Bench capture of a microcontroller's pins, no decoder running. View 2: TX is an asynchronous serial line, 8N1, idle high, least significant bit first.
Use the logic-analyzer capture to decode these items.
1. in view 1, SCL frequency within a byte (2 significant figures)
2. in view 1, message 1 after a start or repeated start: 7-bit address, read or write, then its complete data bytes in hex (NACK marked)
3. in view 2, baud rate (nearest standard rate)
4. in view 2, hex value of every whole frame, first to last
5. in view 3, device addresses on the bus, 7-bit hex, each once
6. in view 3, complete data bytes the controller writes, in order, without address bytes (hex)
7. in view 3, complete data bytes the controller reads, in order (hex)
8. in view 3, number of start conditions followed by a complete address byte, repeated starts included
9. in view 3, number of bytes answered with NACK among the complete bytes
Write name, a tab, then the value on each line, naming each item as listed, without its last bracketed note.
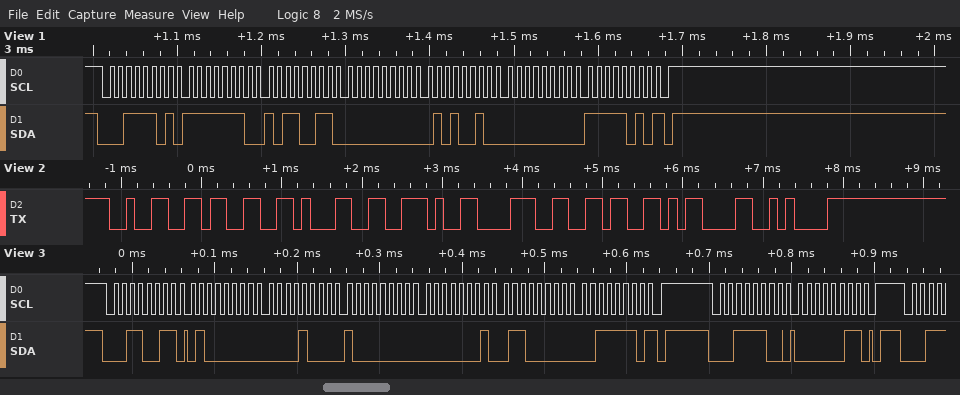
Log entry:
in view 1, SCL frequency within a byte	100 kHz
in view 1, message 1 after a start or repeated start: 7-bit address, read or write, then its complete data bytes in hex	0x1E read: FE B3 00 52 00 FA NACK
in view 2, baud rate	9600 baud
in view 2, hex value of every whole frame, first to last	0x32 0x33 0x31 0x2E 0x38 0x36 0x0D 0x0A
in view 3, device addresses on the bus, 7-bit hex, each once	0x19 0x1E
in view 3, complete data bytes the controller writes, in order, without address bytes	03
in view 3, complete data bytes the controller reads, in order	40 08 80 01 60 3E
in view 3, number of start conditions followed by a complete address byte, repeated starts included	2
in view 3, number of bytes answered with NACK among the complete bytes	1
